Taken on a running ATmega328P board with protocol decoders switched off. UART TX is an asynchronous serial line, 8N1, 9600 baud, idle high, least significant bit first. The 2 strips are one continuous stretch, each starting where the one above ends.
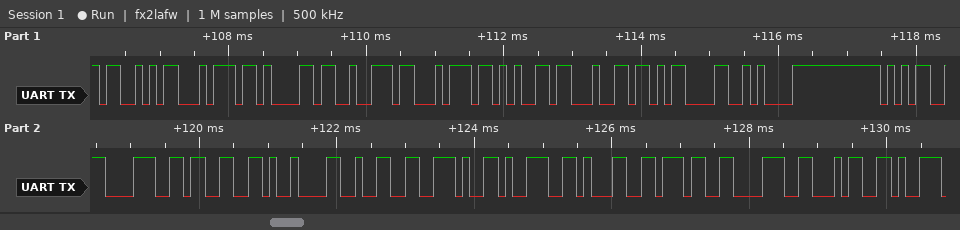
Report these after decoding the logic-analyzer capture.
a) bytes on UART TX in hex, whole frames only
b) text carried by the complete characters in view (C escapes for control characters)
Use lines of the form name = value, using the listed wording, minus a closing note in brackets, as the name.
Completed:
bytes on UART TX in hex, whole frames only = 53 74 61 72 74 65 64 0D 0A 35 38 33 09 32 2E 39 31 37 38 34
text carried by the complete characters in view = "Started\r\n583\t2.91784"
